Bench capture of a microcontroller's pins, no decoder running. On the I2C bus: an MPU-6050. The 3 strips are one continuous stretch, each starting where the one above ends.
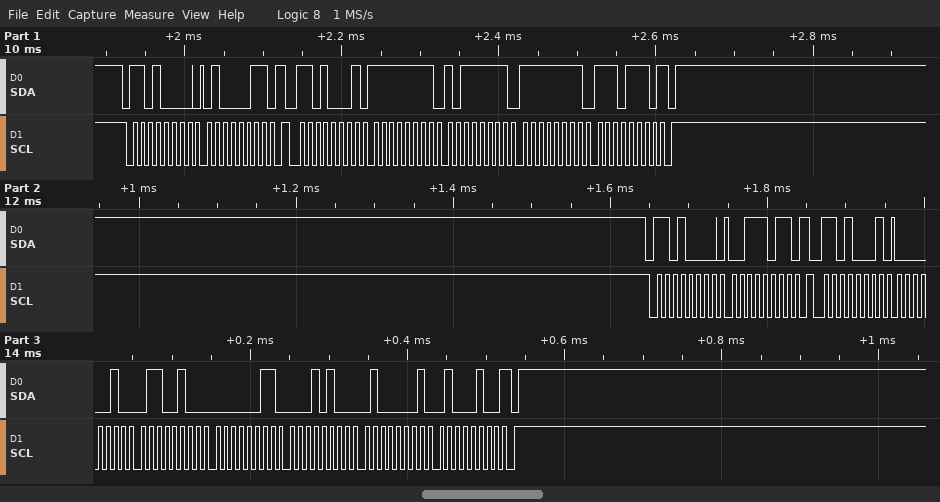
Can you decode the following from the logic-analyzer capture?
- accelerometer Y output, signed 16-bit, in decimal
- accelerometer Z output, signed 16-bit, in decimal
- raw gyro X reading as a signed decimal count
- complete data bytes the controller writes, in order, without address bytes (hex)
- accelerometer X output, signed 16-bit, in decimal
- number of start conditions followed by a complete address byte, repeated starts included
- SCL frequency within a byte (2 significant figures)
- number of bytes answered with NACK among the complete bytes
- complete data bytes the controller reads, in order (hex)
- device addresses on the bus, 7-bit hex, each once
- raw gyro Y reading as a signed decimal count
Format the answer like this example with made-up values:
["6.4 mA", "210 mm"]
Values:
["788", "16708", "-65", "43 3B", "612", "4", "100 kHz", "2", "FF BF FF EE 02 64 03 14 41 44", "0x68", "-18"]
